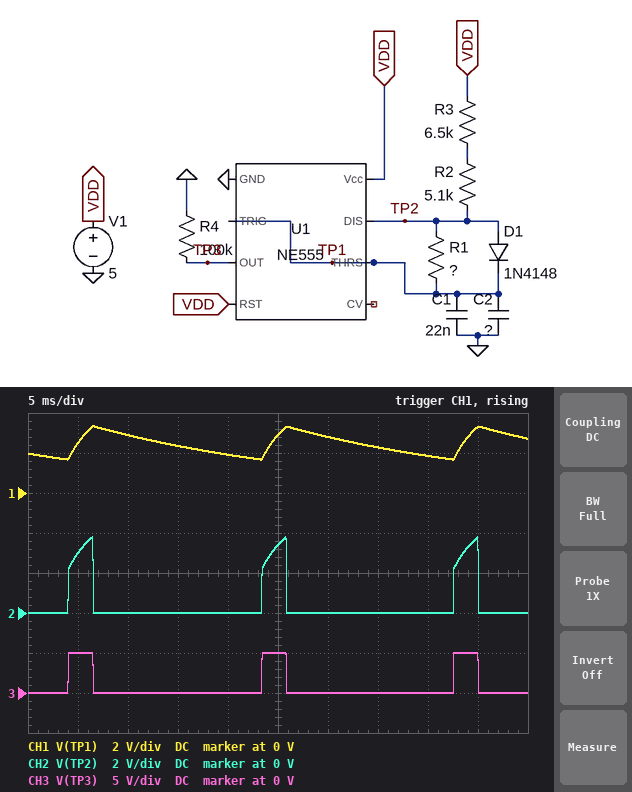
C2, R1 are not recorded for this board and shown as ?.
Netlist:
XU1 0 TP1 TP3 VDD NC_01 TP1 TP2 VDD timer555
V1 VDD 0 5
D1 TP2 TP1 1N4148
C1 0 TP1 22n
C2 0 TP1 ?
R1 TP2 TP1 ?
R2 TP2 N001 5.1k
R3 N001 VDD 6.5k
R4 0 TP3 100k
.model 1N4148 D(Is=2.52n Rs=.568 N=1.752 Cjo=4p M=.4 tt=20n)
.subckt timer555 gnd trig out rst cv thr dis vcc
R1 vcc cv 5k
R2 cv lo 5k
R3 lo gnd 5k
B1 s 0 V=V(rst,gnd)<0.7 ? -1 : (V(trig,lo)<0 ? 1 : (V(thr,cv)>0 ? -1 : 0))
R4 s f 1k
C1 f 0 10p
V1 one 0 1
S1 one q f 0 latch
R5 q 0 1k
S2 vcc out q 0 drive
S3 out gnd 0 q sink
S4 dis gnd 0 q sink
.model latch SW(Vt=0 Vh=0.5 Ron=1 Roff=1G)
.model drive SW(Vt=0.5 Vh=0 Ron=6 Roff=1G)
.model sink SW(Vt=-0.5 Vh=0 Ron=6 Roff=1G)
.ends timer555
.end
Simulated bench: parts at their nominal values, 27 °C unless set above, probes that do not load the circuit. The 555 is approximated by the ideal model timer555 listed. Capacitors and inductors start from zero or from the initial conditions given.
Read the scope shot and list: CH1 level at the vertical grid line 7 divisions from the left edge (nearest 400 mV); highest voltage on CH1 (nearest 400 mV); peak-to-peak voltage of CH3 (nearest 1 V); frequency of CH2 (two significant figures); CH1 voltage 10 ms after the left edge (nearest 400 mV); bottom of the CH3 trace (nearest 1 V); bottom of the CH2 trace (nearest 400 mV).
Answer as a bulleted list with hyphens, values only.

- 2.4 V
- 3.2 V
- 5 V
- 52 Hz
- 2.8 V
- 0 V
- 0 V
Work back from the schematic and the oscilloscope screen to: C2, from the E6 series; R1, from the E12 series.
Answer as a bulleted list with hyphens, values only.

- 220 nF
- 100 kΩ
